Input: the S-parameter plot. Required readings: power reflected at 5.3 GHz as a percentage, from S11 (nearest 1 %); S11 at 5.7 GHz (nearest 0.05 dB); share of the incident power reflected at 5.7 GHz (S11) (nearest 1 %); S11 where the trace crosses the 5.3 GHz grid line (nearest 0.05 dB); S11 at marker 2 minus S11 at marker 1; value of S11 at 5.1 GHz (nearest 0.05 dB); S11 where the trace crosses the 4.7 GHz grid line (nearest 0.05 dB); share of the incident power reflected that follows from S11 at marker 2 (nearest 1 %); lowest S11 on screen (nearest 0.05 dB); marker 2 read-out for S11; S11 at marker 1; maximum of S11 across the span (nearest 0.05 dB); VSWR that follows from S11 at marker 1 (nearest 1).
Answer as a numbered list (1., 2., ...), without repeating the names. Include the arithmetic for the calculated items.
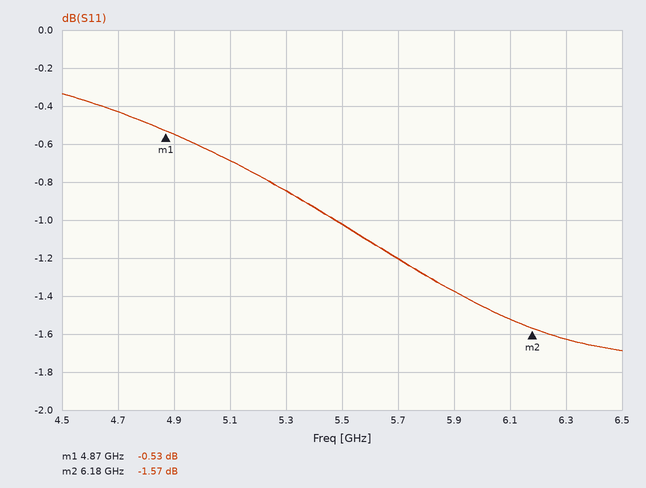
1. 10^(-0.85/10) ≈ 82 %
2. -1.20 dB
3. 10^(-1.2/10) ≈ 76 %
4. -0.85 dB
5. -1.57 − (-0.53) = -1.04 dB
6. -0.70 dB
7. -0.45 dB
8. 10^(-1.57/10) ≈ 70 %
9. -1.70 dB
10. -1.57 dB
11. -0.53 dB
12. -0.35 dB
13. (1 + 0.9408)/(1 − 0.9408) ≈ 33
